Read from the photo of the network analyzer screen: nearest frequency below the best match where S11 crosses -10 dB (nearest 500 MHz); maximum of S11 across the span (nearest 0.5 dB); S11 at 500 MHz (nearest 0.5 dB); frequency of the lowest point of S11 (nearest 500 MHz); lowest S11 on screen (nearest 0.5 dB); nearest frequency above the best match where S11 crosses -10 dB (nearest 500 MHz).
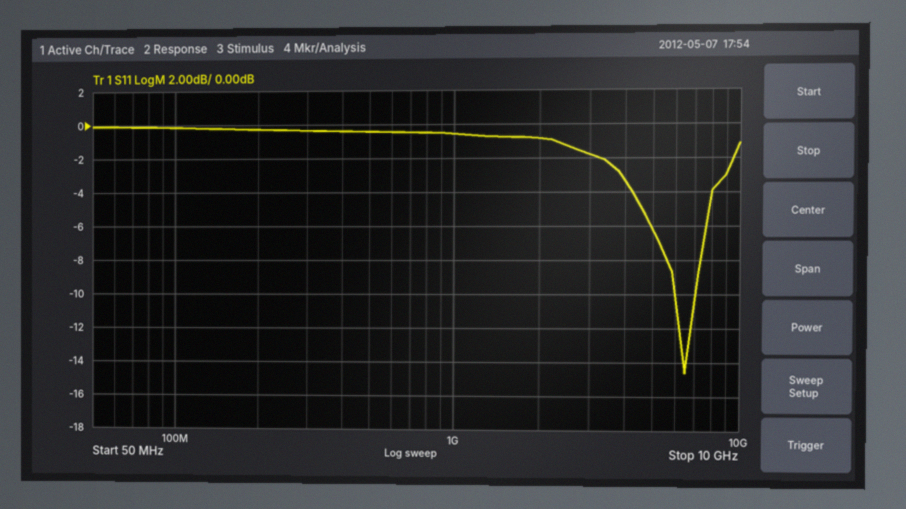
6.0 GHz
0.0 dB
-0.5 dB
6.5 GHz
-14.5 dB
7.0 GHz
